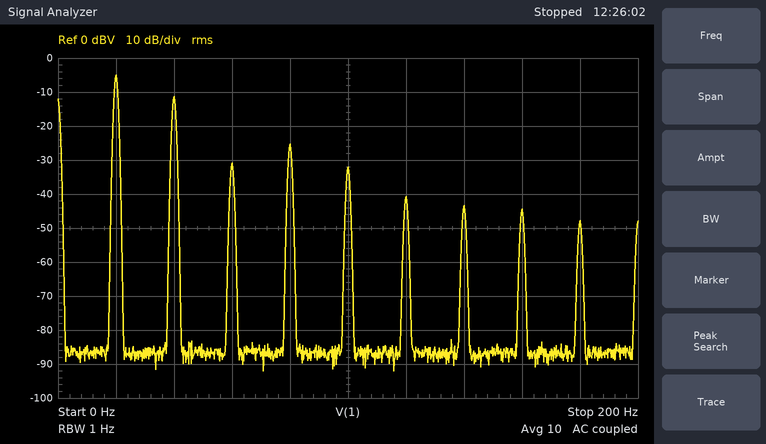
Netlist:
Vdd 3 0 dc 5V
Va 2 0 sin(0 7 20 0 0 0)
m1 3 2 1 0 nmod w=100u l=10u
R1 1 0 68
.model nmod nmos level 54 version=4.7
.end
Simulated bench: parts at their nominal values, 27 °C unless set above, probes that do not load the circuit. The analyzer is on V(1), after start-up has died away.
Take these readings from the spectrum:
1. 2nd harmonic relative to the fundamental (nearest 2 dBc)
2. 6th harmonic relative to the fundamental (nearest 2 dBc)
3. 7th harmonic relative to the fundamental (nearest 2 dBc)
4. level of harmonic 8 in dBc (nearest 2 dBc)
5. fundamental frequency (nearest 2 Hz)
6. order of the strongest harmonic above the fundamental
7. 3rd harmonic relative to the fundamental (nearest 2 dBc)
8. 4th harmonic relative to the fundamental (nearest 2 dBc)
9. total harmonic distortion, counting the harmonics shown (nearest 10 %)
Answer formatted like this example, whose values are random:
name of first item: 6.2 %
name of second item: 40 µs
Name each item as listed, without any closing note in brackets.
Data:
2nd harmonic relative to the fundamental: -6 dBc
6th harmonic relative to the fundamental: -36 dBc
7th harmonic relative to the fundamental: -38 dBc
level of harmonic 8 in dBc: -40 dBc
fundamental frequency: 20 Hz
order of the strongest harmonic above the fundamental: 2
3rd harmonic relative to the fundamental: -26 dBc
4th harmonic relative to the fundamental: -20 dBc
total harmonic distortion, counting the harmonics shown: 50 %
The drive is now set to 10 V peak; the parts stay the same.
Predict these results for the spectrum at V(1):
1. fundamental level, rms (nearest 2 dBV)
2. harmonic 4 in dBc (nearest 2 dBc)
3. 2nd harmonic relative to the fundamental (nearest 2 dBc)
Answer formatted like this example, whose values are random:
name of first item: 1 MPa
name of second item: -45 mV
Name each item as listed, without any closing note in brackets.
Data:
fundamental level, rms: -2 dBV
harmonic 4 in dBc: -16 dBc
2nd harmonic relative to the fundamental: -8 dBc
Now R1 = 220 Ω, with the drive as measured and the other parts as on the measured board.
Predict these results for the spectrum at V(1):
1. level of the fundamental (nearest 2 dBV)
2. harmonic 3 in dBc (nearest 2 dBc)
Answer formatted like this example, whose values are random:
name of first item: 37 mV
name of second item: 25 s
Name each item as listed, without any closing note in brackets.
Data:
level of the fundamental: 0 dBV
harmonic 3 in dBc: -32 dBc
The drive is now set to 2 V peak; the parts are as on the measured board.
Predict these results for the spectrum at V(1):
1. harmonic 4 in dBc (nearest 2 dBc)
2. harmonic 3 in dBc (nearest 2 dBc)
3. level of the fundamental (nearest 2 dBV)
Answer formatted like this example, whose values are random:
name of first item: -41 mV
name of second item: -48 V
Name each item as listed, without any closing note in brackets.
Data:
harmonic 4 in dBc: -26 dBc
harmonic 3 in dBc: -18 dBc
level of the fundamental: -20 dBV
